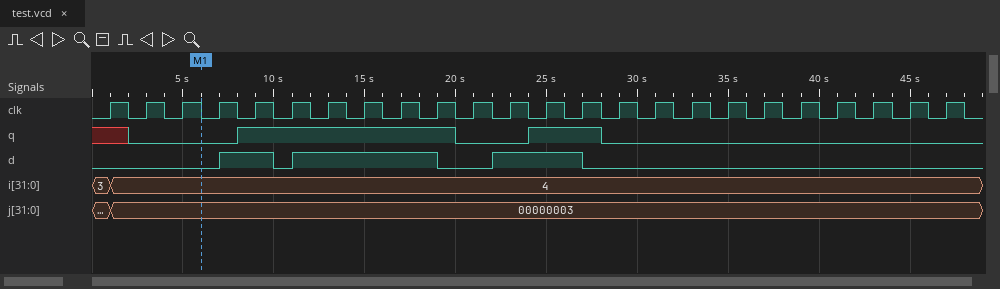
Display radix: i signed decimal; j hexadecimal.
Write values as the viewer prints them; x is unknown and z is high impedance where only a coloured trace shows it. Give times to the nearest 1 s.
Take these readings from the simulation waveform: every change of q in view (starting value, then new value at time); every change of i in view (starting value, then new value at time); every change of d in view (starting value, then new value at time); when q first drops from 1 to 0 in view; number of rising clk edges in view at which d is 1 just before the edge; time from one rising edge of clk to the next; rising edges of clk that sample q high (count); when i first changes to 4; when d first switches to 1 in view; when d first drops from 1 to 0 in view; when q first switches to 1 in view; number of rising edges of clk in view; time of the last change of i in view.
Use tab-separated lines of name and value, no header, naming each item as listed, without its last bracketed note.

every change of q in view	x, 0 at 2 s, 1 at 8 s, 0 at 20 s, 1 at 24 s, 0 at 28 s
every change of i in view	3, 4 at 1 s
every change of d in view	0, 1 at 7 s, 0 at 10 s, 1 at 11 s, 0 at 19 s, 1 at 22 s, 0 at 27 s
when q first drops from 1 to 0 in view	20 s
number of rising clk edges in view at which d is 1 just before the edge	8
time from one rising edge of clk to the next	2 s
rising edges of clk that sample q high	8
when i first changes to 4	1 s
when d first switches to 1 in view	7 s
when d first drops from 1 to 0 in view	10 s
when q first switches to 1 in view	8 s
number of rising edges of clk in view	24
time of the last change of i in view	1 s
